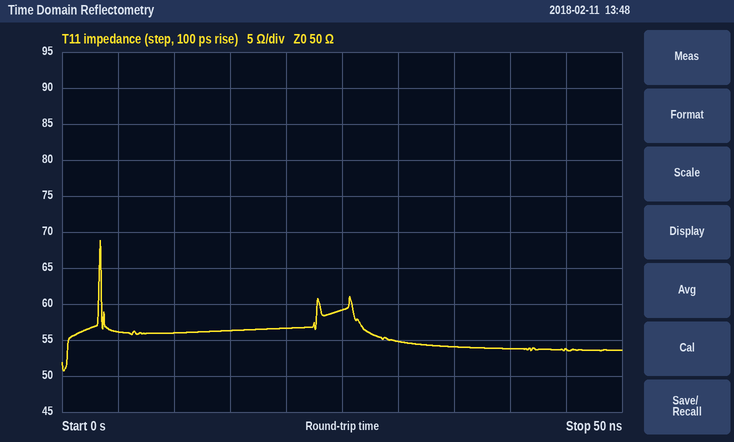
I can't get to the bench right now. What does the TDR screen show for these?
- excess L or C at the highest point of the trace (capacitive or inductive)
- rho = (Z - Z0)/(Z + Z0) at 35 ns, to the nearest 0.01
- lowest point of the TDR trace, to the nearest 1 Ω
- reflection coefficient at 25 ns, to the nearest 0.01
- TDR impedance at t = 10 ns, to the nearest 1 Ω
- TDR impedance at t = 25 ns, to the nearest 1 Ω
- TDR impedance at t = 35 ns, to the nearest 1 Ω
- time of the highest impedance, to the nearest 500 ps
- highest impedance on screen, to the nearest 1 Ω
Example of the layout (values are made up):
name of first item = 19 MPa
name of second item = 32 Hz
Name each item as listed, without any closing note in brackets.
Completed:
excess L or C at the highest point of the trace = inductive
rho = (Z - Z0)/(Z + Z0) at 35 ns, to the nearest 0.01 = +0.04
lowest point of the TDR trace, to the nearest 1 Ω = 51 Ω
reflection coefficient at 25 ns, to the nearest 0.01 = +0.08
TDR impedance at t = 10 ns, to the nearest 1 Ω = 56 Ω
TDR impedance at t = 25 ns, to the nearest 1 Ω = 59 Ω
TDR impedance at t = 35 ns, to the nearest 1 Ω = 54 Ω
time of the highest impedance, to the nearest 500 ps = 3.5 ns
highest impedance on screen, to the nearest 1 Ω = 69 Ω
